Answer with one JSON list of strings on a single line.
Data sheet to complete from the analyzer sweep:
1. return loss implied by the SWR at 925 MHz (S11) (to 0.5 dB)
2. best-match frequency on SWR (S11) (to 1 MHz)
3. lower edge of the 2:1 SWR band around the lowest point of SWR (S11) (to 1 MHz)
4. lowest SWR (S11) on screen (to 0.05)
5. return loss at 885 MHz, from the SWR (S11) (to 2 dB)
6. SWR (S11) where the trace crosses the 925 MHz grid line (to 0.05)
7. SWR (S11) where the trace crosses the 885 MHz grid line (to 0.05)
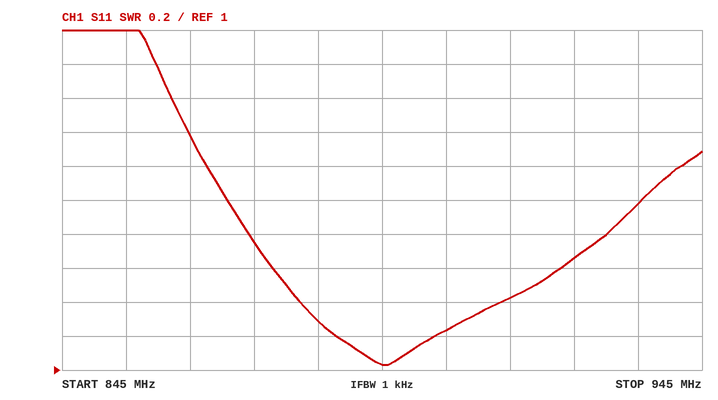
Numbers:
["12.0 dB", "895 MHz", "871 MHz", "1.05", "18 dB", "1.65", "1.30"]
